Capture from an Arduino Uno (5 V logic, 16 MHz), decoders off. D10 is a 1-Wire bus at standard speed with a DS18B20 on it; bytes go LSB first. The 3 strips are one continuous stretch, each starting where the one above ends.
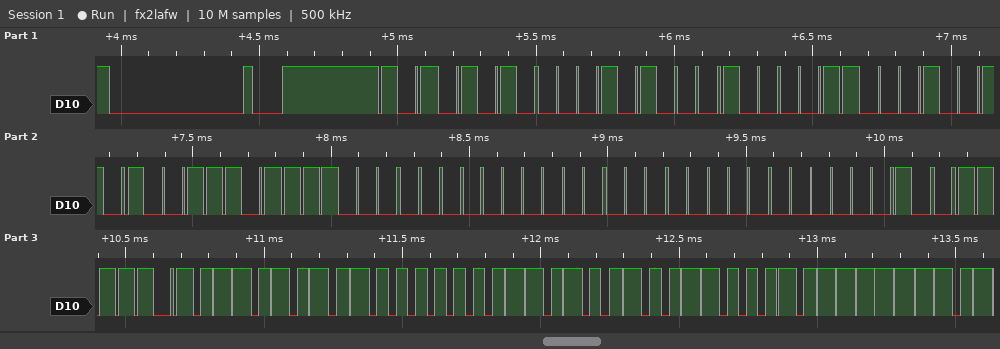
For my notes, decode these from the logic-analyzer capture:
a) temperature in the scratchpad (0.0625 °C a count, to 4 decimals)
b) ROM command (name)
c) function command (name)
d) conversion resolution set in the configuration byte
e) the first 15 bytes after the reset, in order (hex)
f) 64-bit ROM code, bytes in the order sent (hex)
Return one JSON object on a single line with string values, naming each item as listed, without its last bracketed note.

{"temperature in the scratchpad": "21.3750 °C", "ROM command": "Match ROM", "function command": "Read Scratchpad", "conversion resolution set in the configuration byte": "12 bits", "the first 15 bytes after the reset, in order": "55 28 C2 48 B9 07 00 00 40 BE 56 01 4B 46 7F", "64-bit ROM code, bytes in the order sent": "28 C2 48 B9 07 00 00 40"}
